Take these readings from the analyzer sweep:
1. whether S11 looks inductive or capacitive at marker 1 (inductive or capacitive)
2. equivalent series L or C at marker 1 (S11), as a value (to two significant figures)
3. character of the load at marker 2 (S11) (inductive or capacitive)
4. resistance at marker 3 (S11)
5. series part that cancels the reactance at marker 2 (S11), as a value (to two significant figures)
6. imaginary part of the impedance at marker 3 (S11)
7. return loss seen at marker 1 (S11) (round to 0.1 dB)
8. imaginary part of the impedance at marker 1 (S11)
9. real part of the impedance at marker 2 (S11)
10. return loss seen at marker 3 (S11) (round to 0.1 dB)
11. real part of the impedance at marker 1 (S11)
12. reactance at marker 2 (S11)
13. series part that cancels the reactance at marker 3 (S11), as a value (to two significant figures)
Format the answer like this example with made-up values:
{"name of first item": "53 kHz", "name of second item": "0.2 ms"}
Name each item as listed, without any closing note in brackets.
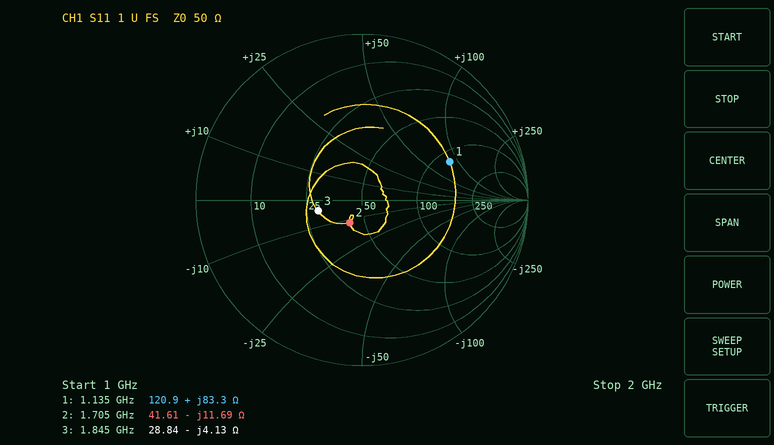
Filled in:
{"whether S11 looks inductive or capacitive at marker 1": "inductive", "equivalent series L or C at marker 1 (S11), as a value": "12 nH", "character of the load at marker 2 (S11)": "capacitive", "resistance at marker 3": "28.84 Ω", "series part that cancels the reactance at marker 2 (S11), as a value": "1.1 nH", "imaginary part of the impedance at marker 3": "-4.13 Ω", "return loss seen at marker 1 (S11)": "4.8 dB", "imaginary part of the impedance at marker 1": "+83.3 Ω", "real part of the impedance at marker 2": "41.61 Ω", "return loss seen at marker 3 (S11)": "11.3 dB", "real part of the impedance at marker 1": "120.9 Ω", "reactance at marker 2": "-11.69 Ω", "series part that cancels the reactance at marker 3 (S11), as a value": "360 pH"}
